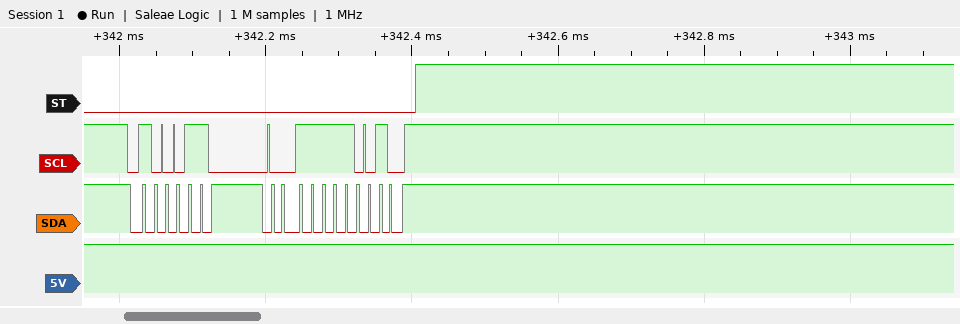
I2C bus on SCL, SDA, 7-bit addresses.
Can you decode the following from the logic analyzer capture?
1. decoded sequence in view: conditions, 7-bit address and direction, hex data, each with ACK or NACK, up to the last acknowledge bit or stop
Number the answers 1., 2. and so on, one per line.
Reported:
1. start, address 46 write ACK, F9 ACK, stop
